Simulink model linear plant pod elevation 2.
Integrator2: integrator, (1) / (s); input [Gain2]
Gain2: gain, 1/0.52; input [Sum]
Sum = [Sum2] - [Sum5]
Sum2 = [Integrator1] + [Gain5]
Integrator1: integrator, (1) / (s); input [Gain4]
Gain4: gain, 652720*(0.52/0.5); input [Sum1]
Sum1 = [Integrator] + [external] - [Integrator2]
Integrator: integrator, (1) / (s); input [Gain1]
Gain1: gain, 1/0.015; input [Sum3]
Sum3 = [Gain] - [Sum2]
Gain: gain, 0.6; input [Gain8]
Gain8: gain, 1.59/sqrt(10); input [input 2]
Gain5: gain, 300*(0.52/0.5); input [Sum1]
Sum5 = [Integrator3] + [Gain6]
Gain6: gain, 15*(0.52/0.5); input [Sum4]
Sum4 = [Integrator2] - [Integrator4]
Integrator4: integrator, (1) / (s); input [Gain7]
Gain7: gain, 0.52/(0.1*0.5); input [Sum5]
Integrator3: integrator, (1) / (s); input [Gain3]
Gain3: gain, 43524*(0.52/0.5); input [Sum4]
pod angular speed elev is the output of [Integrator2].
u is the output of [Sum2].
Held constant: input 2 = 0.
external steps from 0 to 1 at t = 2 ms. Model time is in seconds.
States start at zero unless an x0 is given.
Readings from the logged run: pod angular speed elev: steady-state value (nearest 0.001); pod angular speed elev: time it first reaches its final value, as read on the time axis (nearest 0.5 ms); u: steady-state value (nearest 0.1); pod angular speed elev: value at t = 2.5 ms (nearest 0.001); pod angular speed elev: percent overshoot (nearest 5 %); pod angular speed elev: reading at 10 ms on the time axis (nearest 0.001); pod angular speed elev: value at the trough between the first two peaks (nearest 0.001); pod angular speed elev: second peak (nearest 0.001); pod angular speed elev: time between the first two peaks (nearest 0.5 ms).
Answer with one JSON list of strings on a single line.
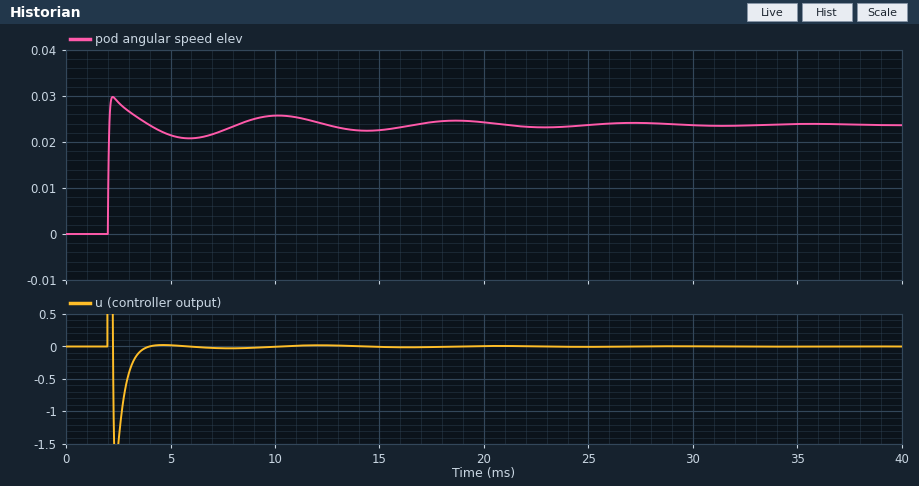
["0.024", "2.0 ms", "0.0", "0.029", "25 %", "0.026", "0.021", "0.026", "8.0 ms"]
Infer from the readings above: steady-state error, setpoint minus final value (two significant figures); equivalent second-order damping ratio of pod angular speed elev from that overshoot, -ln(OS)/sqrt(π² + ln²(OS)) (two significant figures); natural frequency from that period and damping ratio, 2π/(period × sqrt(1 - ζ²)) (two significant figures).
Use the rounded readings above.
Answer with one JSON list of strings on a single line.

["0.98", "0.40", "0.86 rad/ms"]
